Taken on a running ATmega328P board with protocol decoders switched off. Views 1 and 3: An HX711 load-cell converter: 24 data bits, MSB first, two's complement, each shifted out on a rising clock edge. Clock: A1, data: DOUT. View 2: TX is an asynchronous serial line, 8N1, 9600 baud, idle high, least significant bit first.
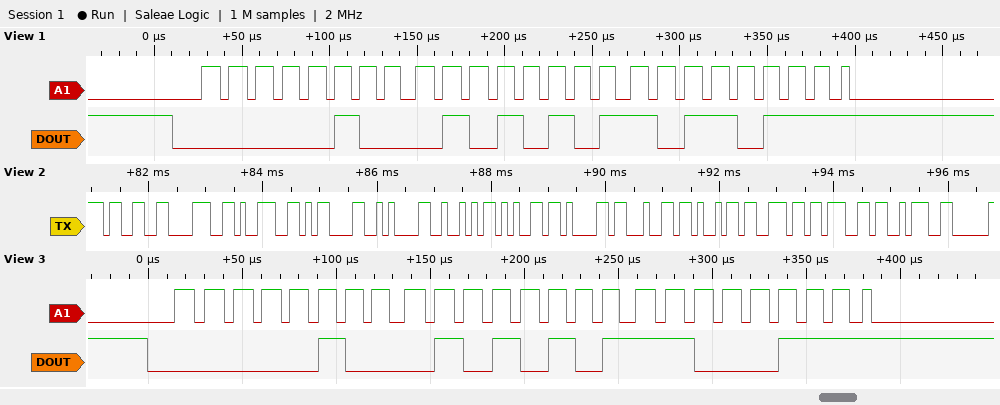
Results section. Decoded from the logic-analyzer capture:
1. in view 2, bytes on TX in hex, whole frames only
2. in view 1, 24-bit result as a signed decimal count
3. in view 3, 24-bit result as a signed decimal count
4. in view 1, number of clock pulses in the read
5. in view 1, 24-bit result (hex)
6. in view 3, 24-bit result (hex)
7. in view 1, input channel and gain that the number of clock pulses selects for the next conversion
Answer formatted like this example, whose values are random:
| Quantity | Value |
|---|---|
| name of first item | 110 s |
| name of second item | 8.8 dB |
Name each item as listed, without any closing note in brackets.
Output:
| Quantity | Value |
|---|---|
| in view 2, bytes on TX in hex, whole frames only | 0x33 0x38 0x39 0x0D 0x0A 0x52 0x65 0x61 0x64 0x69 0x6E 0x67 0x3A |
| in view 1, 24-bit result as a signed decimal count | 284087 |
| in view 3, 24-bit result as a signed decimal count | 284103 |
| in view 1, number of clock pulses in the read | 25 |
| in view 1, 24-bit result | 0x0455B7 |
| in view 3, 24-bit result | 0x0455C7 |
| in view 1, input channel and gain that the number of clock pulses selects for the next conversion | channel A, gain 128 |
